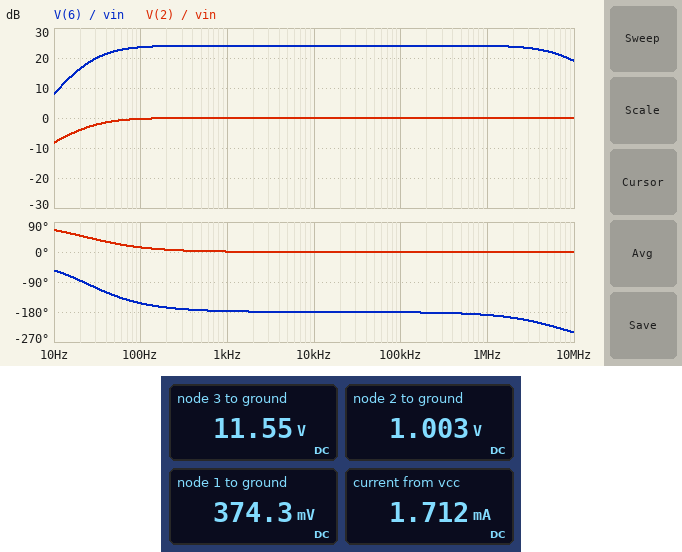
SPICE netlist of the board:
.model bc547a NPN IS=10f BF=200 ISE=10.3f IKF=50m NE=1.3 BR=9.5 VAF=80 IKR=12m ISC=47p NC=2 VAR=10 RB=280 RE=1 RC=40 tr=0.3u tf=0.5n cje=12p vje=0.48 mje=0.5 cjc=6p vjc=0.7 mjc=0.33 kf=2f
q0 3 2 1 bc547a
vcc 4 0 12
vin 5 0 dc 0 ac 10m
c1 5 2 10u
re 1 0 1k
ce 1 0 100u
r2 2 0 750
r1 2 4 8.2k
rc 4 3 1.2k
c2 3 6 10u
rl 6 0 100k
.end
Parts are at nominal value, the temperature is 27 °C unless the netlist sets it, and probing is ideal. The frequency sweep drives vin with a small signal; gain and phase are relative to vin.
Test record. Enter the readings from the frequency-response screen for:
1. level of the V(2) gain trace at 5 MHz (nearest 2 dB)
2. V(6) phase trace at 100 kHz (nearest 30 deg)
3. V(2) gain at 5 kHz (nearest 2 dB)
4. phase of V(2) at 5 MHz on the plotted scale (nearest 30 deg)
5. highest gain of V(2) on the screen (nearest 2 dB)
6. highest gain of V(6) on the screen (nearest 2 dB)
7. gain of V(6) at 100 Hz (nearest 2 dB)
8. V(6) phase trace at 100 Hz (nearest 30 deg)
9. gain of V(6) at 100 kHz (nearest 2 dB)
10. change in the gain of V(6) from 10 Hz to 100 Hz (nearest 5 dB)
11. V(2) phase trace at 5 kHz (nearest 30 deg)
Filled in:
0 dB
-180 deg
0 dB
0 deg
0 dB
24 dB
24 dB
-150 deg
24 dB
15 dB
0 deg
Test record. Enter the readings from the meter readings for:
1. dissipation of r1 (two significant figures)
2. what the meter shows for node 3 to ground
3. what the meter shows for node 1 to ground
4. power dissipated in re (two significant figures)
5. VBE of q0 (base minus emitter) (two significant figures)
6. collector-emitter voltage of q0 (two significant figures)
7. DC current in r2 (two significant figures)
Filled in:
15 mW
11.55 V
374.3 mV
140 µW
630 mV
11 V
1.3 mA
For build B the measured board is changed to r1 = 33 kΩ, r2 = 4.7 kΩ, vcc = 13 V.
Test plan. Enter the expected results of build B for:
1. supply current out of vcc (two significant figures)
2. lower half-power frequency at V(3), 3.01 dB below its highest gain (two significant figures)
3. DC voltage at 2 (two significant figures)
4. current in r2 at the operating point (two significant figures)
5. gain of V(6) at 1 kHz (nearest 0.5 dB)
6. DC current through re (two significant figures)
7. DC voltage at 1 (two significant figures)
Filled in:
1.3 mA
56 Hz
1.6 V
340 µA
31.5 dB
940 µA
940 mV
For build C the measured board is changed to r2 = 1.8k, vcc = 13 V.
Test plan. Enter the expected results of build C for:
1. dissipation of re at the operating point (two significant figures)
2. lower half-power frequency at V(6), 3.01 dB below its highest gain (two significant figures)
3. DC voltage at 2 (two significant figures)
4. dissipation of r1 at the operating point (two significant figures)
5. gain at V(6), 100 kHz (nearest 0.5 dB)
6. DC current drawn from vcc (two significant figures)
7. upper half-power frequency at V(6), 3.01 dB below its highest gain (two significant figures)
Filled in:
2.7 mW
90 Hz
2.3 V
14 mW
35.5 dB
2.9 mA
2.6 MHz
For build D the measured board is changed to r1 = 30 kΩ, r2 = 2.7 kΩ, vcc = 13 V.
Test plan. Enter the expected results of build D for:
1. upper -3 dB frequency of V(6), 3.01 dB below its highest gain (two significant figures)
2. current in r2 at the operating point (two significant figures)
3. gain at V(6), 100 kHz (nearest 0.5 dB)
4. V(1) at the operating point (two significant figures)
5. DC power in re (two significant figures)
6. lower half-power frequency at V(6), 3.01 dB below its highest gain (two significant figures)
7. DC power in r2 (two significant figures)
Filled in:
6.3 MHz
390 µA
25.5 dB
430 mV
190 µW
30 Hz
420 µW
